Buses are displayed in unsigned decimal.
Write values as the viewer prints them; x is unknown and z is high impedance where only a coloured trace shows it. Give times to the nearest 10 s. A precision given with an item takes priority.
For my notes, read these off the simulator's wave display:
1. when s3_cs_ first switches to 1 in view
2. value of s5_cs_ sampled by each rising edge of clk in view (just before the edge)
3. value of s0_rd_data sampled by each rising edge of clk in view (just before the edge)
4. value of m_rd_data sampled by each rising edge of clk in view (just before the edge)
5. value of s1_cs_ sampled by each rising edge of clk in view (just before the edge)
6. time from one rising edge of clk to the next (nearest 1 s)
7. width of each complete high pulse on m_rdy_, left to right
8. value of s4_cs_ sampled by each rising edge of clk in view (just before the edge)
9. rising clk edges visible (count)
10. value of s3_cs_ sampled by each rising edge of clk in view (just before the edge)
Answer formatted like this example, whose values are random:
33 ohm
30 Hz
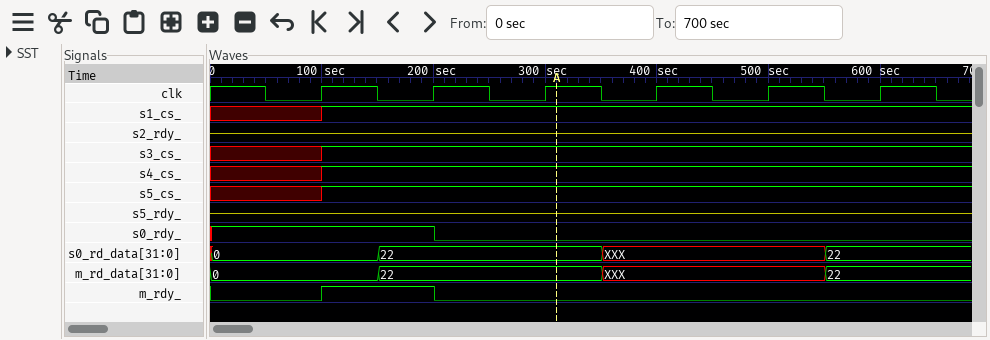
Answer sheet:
100 s
x 1 1 1 1 1
0, 22, 22, XXX, XXX, 22
0, 22, 22, XXX, XXX, 22
x 1 1 1 1 1
100 s
100 s
x 1 1 1 1 1
6
x 1 1 1 1 1
